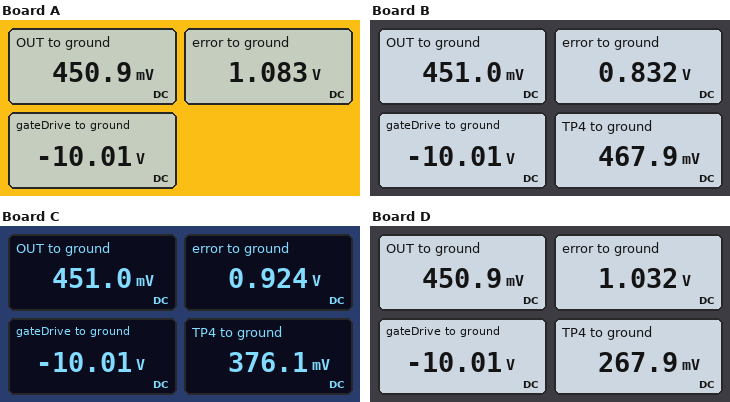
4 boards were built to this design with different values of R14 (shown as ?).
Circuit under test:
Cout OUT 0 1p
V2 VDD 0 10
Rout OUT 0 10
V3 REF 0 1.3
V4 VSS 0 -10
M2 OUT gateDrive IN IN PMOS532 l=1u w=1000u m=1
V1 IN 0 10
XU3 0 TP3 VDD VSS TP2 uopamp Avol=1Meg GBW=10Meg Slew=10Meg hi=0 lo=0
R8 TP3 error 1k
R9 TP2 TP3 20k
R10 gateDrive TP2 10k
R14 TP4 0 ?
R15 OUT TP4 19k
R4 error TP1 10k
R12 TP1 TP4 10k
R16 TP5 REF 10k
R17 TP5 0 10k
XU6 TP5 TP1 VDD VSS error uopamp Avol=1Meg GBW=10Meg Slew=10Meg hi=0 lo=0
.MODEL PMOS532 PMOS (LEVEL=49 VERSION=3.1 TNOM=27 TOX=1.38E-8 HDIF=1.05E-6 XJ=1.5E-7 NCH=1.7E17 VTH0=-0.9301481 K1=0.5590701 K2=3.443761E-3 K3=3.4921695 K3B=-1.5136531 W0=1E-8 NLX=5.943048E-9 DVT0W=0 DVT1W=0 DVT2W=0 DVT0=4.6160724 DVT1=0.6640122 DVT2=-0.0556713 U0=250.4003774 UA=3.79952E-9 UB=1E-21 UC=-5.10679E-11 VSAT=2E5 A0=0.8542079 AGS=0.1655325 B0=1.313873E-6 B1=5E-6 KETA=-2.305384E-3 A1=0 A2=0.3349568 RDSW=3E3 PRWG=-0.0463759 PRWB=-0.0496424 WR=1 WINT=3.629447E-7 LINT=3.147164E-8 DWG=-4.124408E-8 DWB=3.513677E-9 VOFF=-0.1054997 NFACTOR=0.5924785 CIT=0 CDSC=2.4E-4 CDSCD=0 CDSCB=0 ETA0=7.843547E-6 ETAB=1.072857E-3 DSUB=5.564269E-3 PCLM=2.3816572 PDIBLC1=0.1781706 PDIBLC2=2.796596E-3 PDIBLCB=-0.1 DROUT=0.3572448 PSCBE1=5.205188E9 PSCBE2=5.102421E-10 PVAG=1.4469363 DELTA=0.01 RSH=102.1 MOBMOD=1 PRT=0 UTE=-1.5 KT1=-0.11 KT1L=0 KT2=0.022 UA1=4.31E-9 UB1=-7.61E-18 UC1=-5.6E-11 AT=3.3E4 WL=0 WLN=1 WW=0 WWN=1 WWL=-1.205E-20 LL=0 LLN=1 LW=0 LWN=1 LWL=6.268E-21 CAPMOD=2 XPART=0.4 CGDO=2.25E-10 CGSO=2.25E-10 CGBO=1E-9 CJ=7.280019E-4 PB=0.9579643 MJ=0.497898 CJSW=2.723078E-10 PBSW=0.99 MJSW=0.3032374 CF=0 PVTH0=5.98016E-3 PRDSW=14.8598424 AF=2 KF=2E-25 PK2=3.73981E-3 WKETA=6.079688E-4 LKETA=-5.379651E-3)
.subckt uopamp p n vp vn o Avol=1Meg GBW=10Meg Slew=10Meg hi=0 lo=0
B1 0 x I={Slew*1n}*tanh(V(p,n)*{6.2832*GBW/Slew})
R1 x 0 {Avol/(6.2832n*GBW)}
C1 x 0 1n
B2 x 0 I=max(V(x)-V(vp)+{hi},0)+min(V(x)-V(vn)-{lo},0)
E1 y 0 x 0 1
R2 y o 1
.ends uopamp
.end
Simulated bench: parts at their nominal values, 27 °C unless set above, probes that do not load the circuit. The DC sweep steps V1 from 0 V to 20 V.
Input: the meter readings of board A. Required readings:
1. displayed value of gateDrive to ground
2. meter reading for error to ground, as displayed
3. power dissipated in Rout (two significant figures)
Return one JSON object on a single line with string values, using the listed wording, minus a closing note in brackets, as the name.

{"displayed value of gateDrive to ground": "-10.01 V", "meter reading for error to ground, as displayed": "1.083 V", "power dissipated in Rout": "20 mW"}
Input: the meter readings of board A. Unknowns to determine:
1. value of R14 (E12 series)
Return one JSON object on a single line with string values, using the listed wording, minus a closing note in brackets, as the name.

{"value of R14": "3.9 kΩ"}
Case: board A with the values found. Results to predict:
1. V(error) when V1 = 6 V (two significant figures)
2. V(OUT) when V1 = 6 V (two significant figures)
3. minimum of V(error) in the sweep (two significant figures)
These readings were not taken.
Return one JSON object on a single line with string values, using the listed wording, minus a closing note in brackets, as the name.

{"V(error) when V1 = 6 V": "1.1 V", "V(OUT) when V1 = 6 V": "270 mV", "minimum of V(error) in the sweep": "1.0 V"}
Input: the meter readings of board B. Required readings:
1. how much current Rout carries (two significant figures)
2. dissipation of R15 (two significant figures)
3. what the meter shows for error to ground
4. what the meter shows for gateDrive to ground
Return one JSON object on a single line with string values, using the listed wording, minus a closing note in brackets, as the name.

{"how much current Rout carries": "45 mA", "dissipation of R15": "15 nW", "what the meter shows for error to ground": "0.832 V", "what the meter shows for gateDrive to ground": "-10.01 V"}
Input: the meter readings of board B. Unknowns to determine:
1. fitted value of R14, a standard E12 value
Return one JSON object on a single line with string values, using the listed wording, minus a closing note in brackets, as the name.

{"fitted value of R14, a standard E12 value": "27 kΩ"}
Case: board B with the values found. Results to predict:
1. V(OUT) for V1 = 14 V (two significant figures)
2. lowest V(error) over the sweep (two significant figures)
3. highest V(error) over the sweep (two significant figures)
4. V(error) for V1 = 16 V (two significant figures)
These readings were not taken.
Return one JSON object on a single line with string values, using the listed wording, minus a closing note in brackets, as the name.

{"V(OUT) for V1 = 14 V": "630 mV", "lowest V(error) over the sweep": "710 mV", "highest V(error) over the sweep": "960 mV", "V(error) for V1 = 16 V": "760 mV"}
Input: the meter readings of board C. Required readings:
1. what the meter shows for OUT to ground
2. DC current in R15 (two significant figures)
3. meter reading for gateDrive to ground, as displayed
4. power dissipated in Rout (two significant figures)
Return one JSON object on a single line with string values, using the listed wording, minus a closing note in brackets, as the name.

{"what the meter shows for OUT to ground": "451.0 mV", "DC current in R15": "3.9 µA", "meter reading for gateDrive to ground, as displayed": "-10.01 V", "power dissipated in Rout": "20 mW"}
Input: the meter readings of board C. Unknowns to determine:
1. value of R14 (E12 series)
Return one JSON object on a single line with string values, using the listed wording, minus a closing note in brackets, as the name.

{"value of R14": "12 kΩ"}
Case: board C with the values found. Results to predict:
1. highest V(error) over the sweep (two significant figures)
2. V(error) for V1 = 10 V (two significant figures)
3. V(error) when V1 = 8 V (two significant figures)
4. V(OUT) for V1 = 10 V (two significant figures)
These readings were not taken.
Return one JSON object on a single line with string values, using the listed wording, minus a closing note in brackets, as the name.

{"highest V(error) over the sweep": "1.0 V", "V(error) for V1 = 10 V": "920 mV", "V(error) when V1 = 8 V": "940 mV", "V(OUT) for V1 = 10 V": "450 mV"}
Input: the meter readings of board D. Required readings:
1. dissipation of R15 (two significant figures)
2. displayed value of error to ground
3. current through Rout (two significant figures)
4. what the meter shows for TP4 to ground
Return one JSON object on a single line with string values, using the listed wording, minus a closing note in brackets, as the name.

{"dissipation of R15": "1.8 µW", "displayed value of error to ground": "1.032 V", "current through Rout": "45 mA", "what the meter shows for TP4 to ground": "267.9 mV"}
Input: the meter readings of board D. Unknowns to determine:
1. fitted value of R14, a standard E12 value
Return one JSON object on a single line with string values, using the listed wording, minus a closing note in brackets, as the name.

{"fitted value of R14, a standard E12 value": "5.6 kΩ"}
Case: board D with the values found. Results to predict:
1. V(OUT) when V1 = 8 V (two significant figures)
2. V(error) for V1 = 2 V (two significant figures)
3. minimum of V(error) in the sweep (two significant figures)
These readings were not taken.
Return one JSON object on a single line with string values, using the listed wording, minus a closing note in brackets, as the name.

{"V(OUT) when V1 = 8 V": "360 mV", "V(error) for V1 = 2 V": "1.1 V", "minimum of V(error) in the sweep": "960 mV"}
